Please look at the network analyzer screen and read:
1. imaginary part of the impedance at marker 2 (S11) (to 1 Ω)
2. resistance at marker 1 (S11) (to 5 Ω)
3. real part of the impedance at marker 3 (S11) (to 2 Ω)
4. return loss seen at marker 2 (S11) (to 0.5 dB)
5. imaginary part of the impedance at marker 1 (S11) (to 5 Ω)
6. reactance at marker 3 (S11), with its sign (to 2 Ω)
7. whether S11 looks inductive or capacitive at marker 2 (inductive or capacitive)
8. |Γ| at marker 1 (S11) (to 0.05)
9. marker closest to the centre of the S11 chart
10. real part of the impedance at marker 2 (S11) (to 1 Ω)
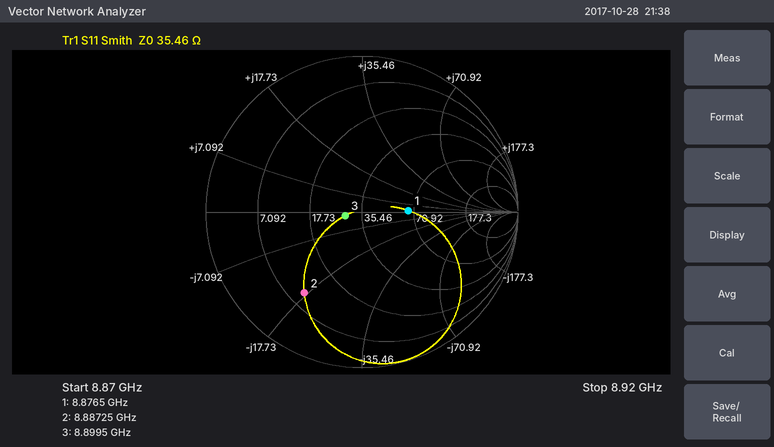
-17 Ω
65 Ω
28 Ω
4.0 dB
0 Ω
-2 Ω
capacitive
0.30
marker 3
10 Ω
